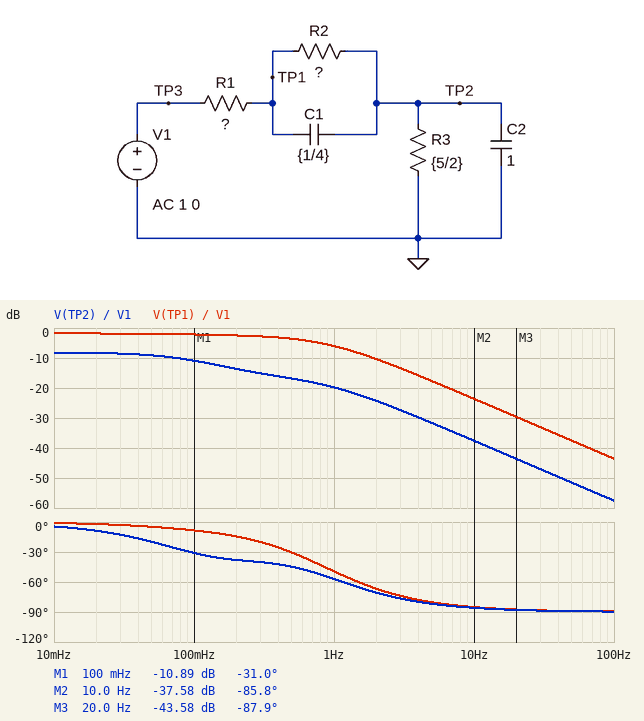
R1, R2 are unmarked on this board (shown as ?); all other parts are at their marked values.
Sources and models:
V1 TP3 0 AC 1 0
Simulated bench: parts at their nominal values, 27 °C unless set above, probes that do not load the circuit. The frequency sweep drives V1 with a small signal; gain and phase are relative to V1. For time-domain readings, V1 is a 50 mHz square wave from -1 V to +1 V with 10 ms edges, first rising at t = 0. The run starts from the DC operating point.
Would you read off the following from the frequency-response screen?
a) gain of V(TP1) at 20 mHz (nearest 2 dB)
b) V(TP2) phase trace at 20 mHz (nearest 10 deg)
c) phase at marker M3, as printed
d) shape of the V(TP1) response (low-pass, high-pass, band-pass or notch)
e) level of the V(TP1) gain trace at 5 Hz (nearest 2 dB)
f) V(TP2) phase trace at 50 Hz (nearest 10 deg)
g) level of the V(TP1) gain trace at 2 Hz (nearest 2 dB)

-2 dB
-10 deg
-87.9 deg
low-pass
-18 dB
-90 deg
-10 dB
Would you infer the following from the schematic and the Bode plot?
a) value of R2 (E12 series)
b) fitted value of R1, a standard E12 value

2.7 Ω
1.2 Ω
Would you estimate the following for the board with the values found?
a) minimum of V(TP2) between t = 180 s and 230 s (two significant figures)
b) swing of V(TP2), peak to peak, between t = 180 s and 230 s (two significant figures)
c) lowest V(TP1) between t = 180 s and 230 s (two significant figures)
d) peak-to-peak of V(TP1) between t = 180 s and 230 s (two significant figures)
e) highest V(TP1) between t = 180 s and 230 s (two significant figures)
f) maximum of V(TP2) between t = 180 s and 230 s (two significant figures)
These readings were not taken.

-390 mV
780 mV
-810 mV
1.6 V
810 mV
390 mV
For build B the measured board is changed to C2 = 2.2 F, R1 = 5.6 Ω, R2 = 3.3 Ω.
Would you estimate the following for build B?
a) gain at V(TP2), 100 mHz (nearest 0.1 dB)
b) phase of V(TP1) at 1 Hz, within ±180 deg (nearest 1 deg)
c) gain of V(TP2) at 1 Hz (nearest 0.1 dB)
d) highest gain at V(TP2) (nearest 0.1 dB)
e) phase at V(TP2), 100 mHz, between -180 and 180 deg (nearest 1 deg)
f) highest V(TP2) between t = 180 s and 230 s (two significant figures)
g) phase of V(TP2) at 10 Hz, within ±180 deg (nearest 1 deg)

-21.9 dB
-73 deg
-38.0 dB
-13.2 dB
-60 deg
180 mV
-89 deg
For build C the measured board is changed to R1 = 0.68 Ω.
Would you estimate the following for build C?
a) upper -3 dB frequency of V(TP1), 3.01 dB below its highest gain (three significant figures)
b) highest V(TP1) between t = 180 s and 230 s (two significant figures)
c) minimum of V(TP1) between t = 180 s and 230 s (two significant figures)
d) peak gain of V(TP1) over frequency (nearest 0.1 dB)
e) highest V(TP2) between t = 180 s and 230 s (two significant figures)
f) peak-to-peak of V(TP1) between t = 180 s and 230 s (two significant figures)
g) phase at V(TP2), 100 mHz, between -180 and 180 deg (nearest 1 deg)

1.27 Hz
880 mV
-880 mV
-1.1 dB
420 mV
1.8 V
-28 deg
